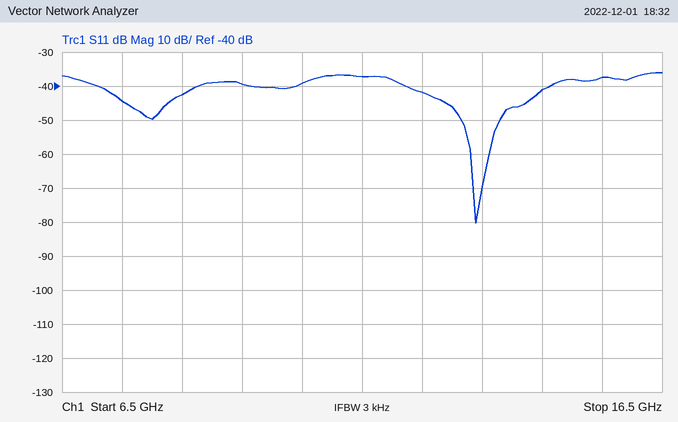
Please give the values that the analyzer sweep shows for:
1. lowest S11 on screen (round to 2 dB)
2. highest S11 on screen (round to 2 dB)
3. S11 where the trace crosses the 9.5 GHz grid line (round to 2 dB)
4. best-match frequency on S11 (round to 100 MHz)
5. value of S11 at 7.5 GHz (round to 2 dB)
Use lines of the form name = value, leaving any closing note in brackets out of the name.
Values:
lowest S11 on screen = -80 dB
highest S11 on screen = -36 dB
S11 where the trace crosses the 9.5 GHz grid line = -40 dB
best-match frequency on S11 = 13.4 GHz
value of S11 at 7.5 GHz = -44 dB
